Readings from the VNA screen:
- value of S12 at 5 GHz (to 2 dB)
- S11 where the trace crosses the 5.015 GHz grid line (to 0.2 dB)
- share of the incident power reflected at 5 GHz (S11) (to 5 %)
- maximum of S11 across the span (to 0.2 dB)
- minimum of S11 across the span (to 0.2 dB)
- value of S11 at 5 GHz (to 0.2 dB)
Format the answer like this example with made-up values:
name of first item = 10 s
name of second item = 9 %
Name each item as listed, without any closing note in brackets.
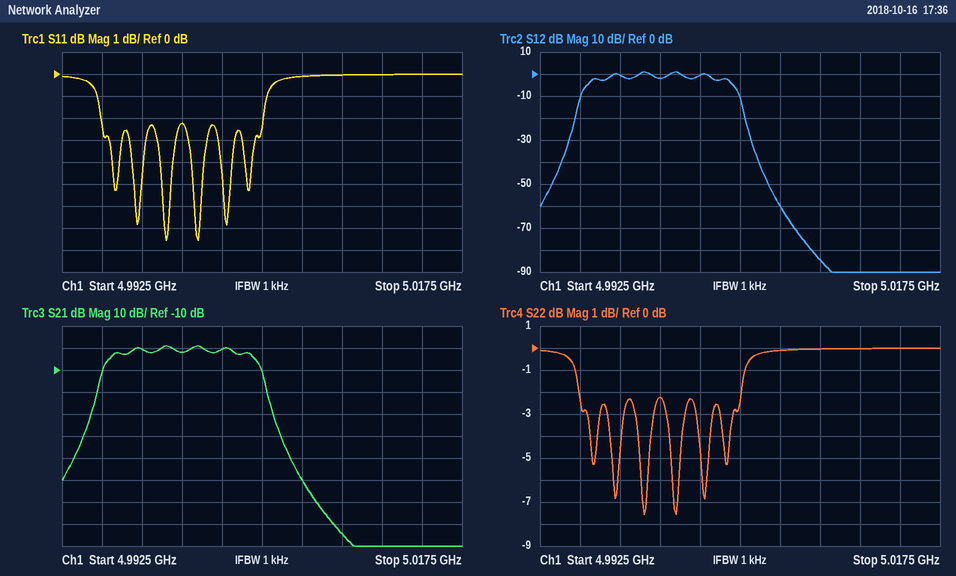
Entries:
value of S12 at 5 GHz = -2 dB
S11 where the trace crosses the 5.015 GHz grid line = 0.0 dB
share of the incident power reflected at 5 GHz (S11) = 60 %
maximum of S11 across the span = 0.0 dB
minimum of S11 across the span = -7.6 dB
value of S11 at 5 GHz = -2.2 dB
